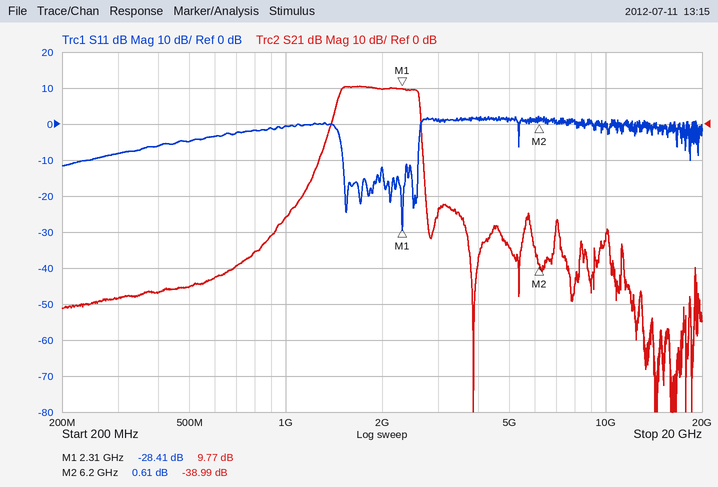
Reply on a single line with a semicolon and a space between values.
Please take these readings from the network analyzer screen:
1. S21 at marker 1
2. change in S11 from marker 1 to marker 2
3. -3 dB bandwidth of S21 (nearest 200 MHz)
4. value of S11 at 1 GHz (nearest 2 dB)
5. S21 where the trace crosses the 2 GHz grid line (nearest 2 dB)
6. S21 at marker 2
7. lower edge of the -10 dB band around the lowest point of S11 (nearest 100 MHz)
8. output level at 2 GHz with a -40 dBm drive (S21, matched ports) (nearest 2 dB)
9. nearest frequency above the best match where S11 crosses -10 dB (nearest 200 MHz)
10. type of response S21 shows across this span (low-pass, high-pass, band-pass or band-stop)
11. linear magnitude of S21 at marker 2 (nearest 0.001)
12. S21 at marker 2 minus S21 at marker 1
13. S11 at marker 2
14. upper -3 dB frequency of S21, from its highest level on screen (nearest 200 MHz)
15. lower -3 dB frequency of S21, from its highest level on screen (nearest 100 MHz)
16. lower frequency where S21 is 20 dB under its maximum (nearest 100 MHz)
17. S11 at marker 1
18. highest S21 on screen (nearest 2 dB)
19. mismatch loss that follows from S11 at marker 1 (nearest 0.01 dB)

9.77 dB; 29.02 dB; 1.2 GHz; 0 dB; 10 dB; -38.99 dB; 1.5 GHz; -30 dBm; 2.6 GHz; band-pass; 0.011; -48.76 dB; 0.61 dB; 2.6 GHz; 1.5 GHz; 1.3 GHz; -28.41 dB; 10 dB; 0.01 dB
